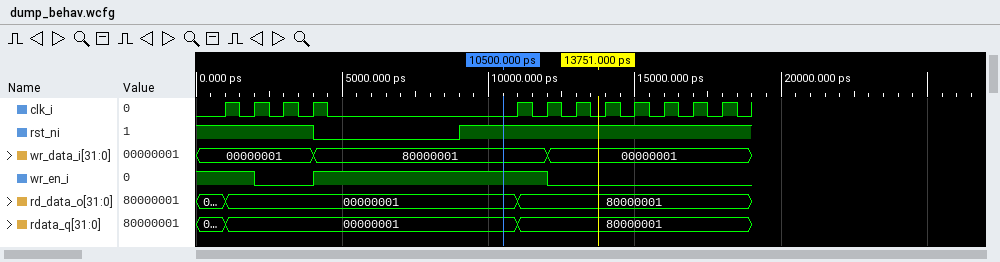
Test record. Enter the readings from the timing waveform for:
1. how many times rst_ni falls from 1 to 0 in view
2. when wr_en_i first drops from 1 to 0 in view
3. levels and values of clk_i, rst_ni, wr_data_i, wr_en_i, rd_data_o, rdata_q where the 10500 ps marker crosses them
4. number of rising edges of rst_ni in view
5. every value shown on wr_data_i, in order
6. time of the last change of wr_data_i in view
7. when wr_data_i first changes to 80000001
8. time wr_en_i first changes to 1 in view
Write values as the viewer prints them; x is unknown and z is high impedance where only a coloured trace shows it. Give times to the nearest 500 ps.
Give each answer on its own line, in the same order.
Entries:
1
2000 ps
clk_i=0, rst_ni=1, wr_data_i=80000001, wr_en_i=1, rd_data_o=00000001, rdata_q=00000001
1
00000001, 80000001, 00000001
12000 ps
4000 ps
4000 ps
